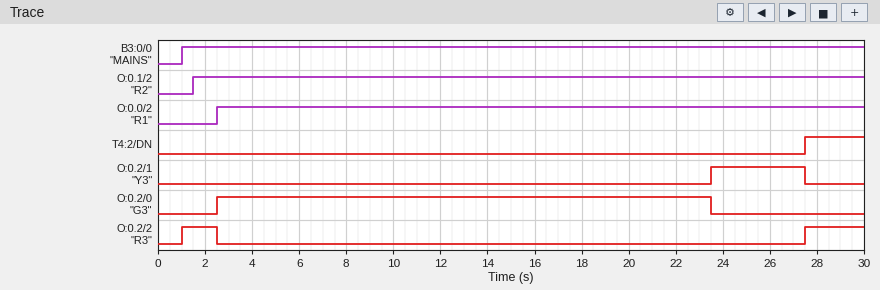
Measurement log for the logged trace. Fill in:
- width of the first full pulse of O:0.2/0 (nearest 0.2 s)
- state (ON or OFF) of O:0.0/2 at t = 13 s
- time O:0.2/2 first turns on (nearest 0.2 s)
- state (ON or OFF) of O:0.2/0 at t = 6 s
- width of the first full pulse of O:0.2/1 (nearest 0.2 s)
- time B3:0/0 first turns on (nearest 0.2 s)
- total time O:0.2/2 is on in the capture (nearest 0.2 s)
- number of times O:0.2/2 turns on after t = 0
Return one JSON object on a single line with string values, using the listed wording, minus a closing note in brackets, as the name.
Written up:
{"width of the first full pulse of O:0.2/0": "21.0 s", "state (ON or OFF) of O:0.0/2 at t = 13 s": "ON", "time O:0.2/2 first turns on": "1.0 s", "state (ON or OFF) of O:0.2/0 at t = 6 s": "ON", "width of the first full pulse of O:0.2/1": "4.0 s", "time B3:0/0 first turns on": "1.0 s", "total time O:0.2/2 is on in the capture": "4.0 s", "number of times O:0.2/2 turns on after t = 0": "2"}
